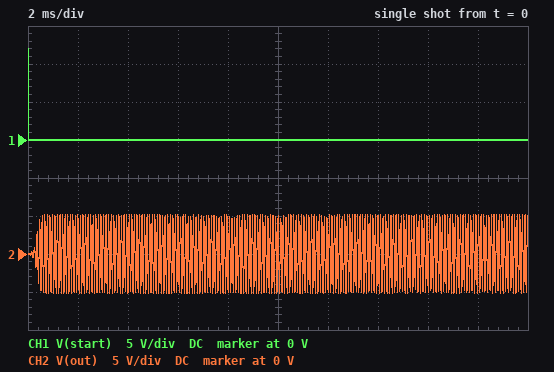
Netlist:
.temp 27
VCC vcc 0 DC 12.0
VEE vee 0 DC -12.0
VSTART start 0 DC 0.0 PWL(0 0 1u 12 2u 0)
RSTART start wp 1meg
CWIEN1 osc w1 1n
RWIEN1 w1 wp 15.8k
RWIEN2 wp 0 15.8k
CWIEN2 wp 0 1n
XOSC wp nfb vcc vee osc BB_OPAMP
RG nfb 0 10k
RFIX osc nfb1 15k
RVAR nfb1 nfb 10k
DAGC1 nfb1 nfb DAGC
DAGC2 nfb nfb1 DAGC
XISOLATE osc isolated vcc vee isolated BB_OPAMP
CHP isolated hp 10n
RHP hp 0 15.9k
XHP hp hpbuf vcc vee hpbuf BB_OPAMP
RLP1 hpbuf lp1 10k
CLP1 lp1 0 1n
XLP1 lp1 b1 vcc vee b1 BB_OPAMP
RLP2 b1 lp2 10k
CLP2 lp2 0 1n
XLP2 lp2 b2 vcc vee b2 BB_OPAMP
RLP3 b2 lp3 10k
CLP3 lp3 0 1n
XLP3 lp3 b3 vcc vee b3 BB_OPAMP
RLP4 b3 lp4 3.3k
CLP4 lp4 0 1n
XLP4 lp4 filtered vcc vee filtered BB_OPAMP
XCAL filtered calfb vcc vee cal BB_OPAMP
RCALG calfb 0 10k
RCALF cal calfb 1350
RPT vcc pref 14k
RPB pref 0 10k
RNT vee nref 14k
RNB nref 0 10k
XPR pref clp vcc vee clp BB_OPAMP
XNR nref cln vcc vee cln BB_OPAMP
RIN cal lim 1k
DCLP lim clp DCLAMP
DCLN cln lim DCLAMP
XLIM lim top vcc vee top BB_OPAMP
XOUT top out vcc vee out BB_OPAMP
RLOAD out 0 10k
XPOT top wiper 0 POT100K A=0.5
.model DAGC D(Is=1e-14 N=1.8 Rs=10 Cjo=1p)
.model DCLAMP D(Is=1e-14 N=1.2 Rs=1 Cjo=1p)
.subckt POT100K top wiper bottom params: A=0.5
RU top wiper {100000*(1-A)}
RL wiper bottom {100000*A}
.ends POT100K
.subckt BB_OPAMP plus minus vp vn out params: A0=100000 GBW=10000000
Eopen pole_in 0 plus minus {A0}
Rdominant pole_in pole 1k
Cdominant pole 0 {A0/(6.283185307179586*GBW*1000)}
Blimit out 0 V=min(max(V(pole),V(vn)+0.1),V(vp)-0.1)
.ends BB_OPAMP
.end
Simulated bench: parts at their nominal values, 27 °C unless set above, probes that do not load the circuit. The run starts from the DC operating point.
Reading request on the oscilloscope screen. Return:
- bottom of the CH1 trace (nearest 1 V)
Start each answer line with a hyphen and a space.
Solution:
- 0 V
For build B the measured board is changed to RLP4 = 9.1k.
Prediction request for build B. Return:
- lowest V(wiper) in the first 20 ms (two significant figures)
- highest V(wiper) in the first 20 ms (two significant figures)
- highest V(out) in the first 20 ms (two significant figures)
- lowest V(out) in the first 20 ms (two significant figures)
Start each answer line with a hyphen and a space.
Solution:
- -2.3 V
- 2.3 V
- 4.6 V
- -4.6 V
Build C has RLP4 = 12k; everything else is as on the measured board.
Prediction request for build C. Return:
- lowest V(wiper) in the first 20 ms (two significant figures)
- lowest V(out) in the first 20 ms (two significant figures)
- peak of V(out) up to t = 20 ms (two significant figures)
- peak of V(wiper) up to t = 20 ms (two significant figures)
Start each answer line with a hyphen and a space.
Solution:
- -2.1 V
- -4.2 V
- 4.2 V
- 2.1 V
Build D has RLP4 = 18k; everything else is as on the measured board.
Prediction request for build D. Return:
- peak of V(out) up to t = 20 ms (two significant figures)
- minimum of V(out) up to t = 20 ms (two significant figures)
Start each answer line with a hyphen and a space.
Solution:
- 3.5 V
- -3.5 V
